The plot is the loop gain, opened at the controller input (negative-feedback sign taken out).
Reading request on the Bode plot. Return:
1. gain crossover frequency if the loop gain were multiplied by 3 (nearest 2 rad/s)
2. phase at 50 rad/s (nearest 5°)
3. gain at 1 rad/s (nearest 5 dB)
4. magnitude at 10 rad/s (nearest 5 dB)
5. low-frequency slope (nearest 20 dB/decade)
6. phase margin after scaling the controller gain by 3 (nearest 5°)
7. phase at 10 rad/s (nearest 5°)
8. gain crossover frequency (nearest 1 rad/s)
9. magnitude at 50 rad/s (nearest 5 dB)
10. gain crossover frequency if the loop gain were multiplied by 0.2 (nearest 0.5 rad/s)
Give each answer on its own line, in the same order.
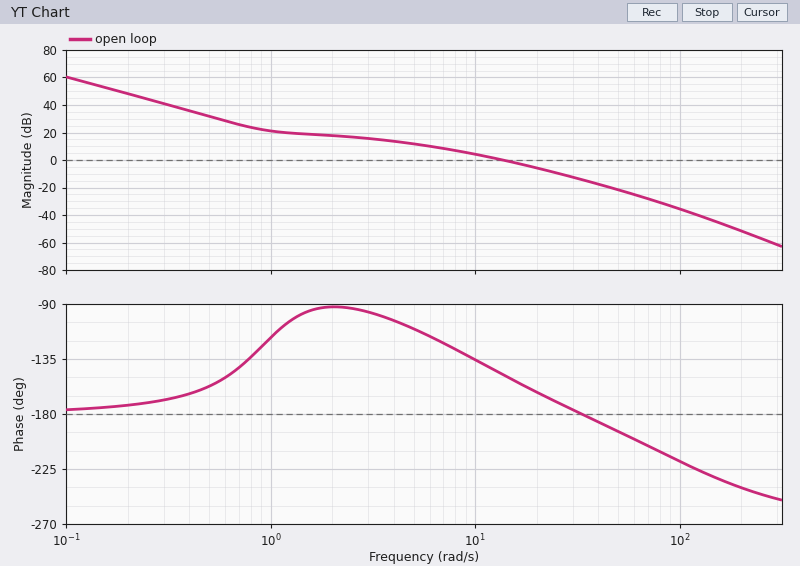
26 rad/s
-195°
20 dB
5 dB
-40 dB/decade
10°
-135°
14 rad/s
-20 dB
4.0 rad/s
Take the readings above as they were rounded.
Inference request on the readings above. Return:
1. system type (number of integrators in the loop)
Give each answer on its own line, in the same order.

2
